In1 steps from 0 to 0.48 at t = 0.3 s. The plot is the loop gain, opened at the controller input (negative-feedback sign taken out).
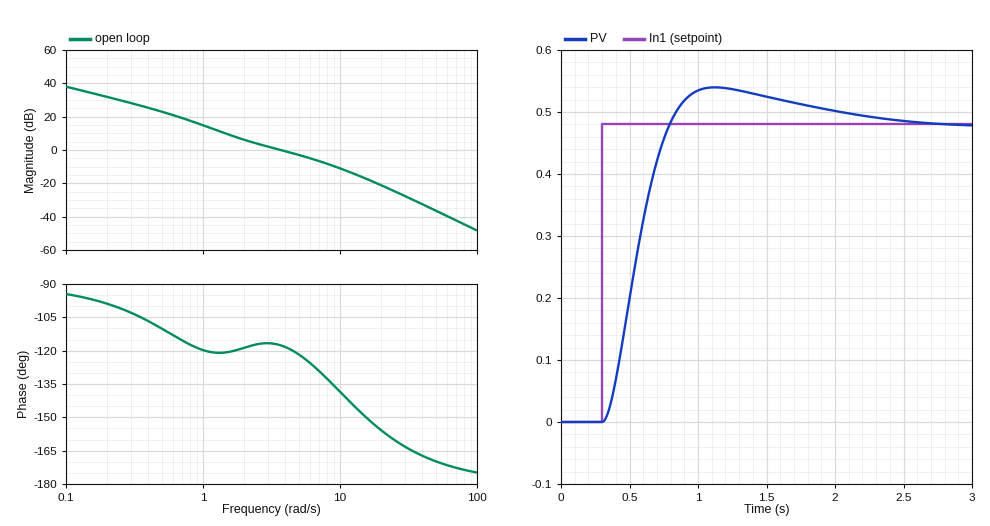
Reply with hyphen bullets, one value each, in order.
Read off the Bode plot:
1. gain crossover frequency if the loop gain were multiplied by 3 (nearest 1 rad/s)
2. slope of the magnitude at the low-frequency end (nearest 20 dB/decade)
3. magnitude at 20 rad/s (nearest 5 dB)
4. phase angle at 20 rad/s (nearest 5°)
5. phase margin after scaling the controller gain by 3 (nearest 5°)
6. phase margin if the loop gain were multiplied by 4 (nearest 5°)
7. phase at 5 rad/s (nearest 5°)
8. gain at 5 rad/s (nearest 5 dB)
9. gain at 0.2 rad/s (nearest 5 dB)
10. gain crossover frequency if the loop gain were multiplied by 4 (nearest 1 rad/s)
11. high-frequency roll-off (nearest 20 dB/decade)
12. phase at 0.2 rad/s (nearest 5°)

- 9 rad/s
- -20 dB/decade
- -20 dB
- -155°
- 45°
- 40°
- -120°
- -5 dB
- 30 dB
- 11 rad/s
- -40 dB/decade
- -100°
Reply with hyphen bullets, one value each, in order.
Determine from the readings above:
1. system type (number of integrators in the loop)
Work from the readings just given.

- 1
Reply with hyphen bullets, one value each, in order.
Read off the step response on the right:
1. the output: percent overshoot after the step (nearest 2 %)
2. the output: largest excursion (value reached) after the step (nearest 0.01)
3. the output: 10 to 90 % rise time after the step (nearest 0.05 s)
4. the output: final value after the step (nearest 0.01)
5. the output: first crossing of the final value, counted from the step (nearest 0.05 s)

- 12 %
- 0.54
- 0.35 s
- 0.48
- 0.50 s
